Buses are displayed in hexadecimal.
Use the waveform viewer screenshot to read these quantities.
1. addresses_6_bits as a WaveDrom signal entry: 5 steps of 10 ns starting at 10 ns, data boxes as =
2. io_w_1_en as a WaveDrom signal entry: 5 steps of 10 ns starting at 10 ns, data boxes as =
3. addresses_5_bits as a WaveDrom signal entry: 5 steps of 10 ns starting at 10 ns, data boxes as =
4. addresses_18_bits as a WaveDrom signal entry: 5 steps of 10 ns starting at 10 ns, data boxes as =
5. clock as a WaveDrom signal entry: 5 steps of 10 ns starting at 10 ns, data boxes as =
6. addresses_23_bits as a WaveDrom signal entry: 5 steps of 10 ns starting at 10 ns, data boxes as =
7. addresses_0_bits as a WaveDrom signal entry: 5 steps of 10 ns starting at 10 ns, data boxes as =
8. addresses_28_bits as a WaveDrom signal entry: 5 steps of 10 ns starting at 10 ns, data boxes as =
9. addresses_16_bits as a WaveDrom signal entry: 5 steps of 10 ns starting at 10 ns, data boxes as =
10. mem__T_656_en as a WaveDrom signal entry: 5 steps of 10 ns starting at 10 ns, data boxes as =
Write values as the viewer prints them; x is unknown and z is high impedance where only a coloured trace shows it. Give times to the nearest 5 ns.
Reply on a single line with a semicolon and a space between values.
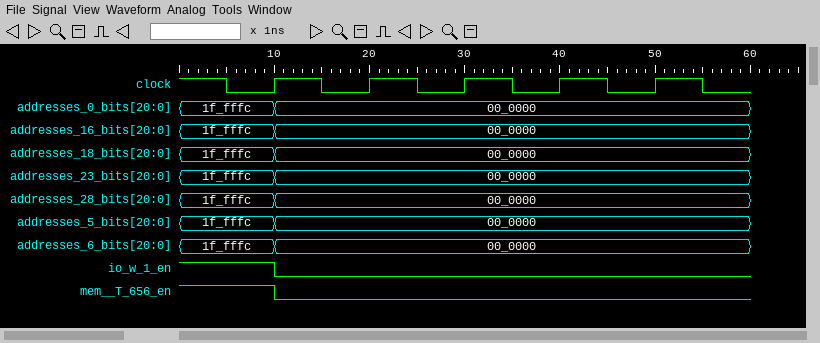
{name: 'addresses_6_bits', wave: '=....', data: '00_0000'}; {name: 'io_w_1_en', wave: '0....'}; {name: 'addresses_5_bits', wave: '=....', data: '00_0000'}; {name: 'addresses_18_bits', wave: '=....', data: '00_0000'}; {name: 'clock', wave: 'p....'}; {name: 'addresses_23_bits', wave: '=....', data: '00_0000'}; {name: 'addresses_0_bits', wave: '=....', data: '00_0000'}; {name: 'addresses_28_bits', wave: '=....', data: '00_0000'}; {name: 'addresses_16_bits', wave: '=....', data: '00_0000'}; {name: 'mem__T_656_en', wave: '0....'}
